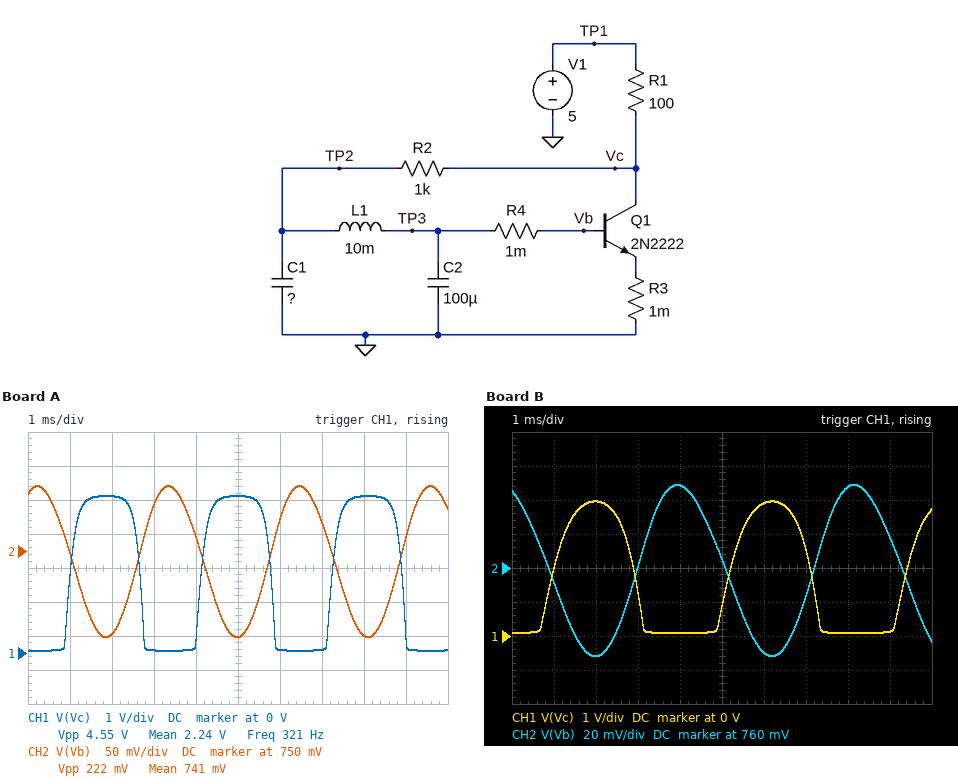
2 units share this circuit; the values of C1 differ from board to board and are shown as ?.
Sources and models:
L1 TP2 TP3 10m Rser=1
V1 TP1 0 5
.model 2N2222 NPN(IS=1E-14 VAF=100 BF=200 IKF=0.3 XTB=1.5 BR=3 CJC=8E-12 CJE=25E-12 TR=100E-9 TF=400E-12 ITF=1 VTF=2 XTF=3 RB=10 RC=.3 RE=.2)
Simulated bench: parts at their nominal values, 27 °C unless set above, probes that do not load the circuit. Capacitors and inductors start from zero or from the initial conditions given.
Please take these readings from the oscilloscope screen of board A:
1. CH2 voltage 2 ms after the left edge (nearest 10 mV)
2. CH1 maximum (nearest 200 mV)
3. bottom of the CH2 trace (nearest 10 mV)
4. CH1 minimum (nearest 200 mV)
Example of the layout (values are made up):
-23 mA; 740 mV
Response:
630 mV; 4.6 V; 620 mV; 0 V
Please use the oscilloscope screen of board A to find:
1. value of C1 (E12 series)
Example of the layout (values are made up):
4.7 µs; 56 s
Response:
33 µF
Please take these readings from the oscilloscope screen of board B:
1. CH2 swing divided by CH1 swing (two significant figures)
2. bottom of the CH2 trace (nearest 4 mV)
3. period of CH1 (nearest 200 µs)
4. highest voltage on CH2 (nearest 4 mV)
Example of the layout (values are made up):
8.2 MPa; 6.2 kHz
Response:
0.026; 708 mV; 4.2 ms; 808 mV
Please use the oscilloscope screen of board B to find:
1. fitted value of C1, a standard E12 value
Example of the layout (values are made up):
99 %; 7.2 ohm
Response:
82 µF
